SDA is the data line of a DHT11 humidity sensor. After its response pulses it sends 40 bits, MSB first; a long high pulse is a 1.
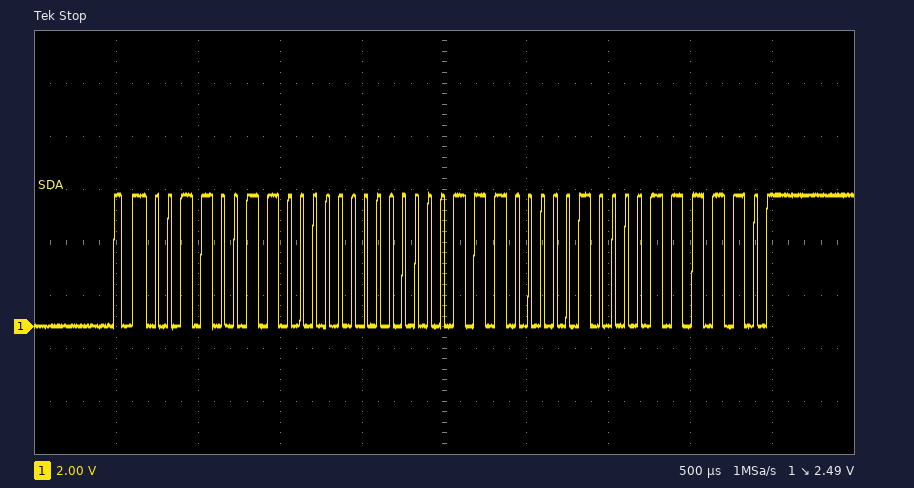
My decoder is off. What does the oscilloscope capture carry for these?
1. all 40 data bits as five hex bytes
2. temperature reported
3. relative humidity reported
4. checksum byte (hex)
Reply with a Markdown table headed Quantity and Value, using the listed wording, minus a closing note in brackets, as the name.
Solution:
| Quantity | Value |
|---|---|
| all 40 data bits as five hex bytes | 33 00 07 04 3E |
| temperature reported | 7.4 °C |
| relative humidity reported | 51 % |
| checksum byte | 0x3E |
